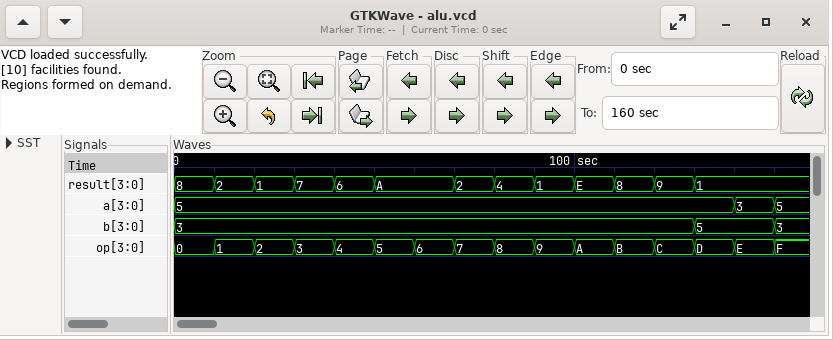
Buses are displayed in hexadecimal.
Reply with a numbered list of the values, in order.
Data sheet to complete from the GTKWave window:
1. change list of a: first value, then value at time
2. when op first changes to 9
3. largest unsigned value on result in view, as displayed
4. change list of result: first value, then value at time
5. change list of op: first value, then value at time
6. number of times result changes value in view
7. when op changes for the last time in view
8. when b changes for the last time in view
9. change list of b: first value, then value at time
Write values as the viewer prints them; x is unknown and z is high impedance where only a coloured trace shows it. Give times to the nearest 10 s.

1. 5, 3 at 140 s, 5 at 150 s
2. 90 s
3. E
4. 8, 2 at 10 s, 1 at 20 s, 7 at 30 s, 6 at 40 s, A at 50 s, 2 at 70 s, 4 at 80 s, 1 at 90 s, E at 100 s, 8 at 110 s, 9 at 120 s, 1 at 130 s
5. 0, 1 at 10 s, 2 at 20 s, 3 at 30 s, 4 at 40 s, 5 at 50 s, 6 at 60 s, 7 at 70 s, 8 at 80 s, 9 at 90 s, A at 100 s, B at 110 s, C at 120 s, D at 130 s, E at 140 s, F at 150 s
6. 12
7. 150 s
8. 150 s
9. 3, 5 at 130 s, 3 at 150 s
